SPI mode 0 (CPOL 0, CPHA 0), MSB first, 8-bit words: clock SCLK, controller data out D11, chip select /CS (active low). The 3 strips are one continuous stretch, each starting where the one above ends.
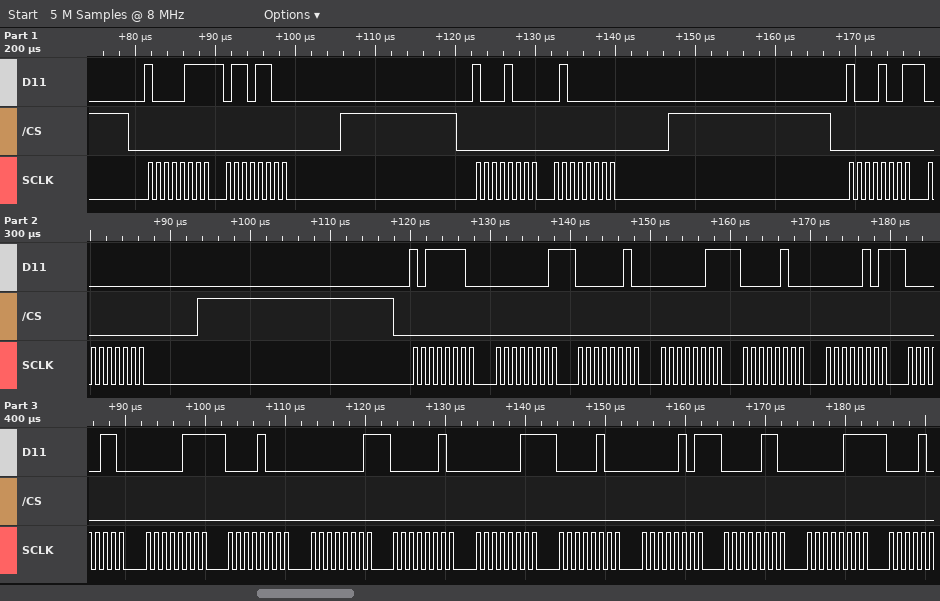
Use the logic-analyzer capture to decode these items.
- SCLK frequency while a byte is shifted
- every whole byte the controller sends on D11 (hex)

1 MHz
0x87 0x6C 0x88 0x40 0x89 0x00 0xBE 0x01 0x02 0x03 0x04 0x05 0x06 0x07 0x08 0x01 0x02 0x03 0x04 0x05 0x06 0x07
